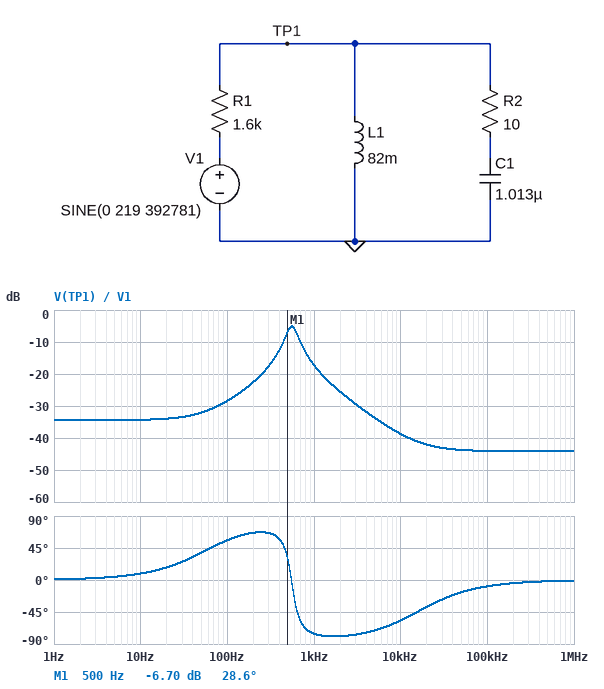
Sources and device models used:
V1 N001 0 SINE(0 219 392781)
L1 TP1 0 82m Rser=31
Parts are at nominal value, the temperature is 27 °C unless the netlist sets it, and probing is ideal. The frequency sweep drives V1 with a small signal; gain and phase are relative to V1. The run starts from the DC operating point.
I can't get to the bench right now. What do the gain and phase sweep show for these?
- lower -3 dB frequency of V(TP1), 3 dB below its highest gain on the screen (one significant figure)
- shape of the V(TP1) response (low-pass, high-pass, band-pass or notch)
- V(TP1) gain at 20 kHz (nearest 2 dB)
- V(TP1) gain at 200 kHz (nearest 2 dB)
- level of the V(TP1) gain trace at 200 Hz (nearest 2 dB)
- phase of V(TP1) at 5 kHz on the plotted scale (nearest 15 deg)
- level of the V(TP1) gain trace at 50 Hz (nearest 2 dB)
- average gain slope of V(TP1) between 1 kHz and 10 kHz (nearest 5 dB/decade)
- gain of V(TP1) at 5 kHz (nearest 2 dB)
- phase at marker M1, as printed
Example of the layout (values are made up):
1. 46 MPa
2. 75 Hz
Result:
1. 500 Hz
2. band-pass
3. -42 dB
4. -44 dB
5. -22 dB
6. -75 deg
7. -32 dB
8. -20 dB/decade
9. -34 dB
10. 28.6 deg
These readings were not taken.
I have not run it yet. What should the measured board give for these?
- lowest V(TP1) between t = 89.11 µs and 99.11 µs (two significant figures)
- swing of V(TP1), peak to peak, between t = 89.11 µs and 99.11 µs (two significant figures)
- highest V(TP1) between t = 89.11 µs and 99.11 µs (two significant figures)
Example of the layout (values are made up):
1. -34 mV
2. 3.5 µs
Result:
1. -1.3 V
2. 2.7 V
3. 1.4 V
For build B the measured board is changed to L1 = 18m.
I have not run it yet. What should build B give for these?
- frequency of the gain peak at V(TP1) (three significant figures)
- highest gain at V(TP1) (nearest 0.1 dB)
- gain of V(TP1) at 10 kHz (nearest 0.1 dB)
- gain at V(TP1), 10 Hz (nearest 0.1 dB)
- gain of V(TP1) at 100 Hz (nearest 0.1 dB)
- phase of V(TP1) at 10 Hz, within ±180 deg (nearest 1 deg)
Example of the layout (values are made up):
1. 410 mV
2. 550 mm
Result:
1. 1.18 kHz
2. -13.2 dB
3. -38.6 dB
4. -34.4 dB
5. -33.8 dB
6. 2 deg
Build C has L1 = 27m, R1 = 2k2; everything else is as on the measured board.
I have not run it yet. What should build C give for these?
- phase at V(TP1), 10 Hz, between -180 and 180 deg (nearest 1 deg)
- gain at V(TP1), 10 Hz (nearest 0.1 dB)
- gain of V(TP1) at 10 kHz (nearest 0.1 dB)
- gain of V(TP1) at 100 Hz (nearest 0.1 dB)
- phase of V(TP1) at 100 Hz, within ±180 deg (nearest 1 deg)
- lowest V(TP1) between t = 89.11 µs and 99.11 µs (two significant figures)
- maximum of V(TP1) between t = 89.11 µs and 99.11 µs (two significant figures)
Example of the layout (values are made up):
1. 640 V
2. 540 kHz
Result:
1. 3 deg
2. -37.1 dB
3. -41.4 dB
4. -35.9 dB
5. 27 deg
6. -960 mV
7. 1.0 V
